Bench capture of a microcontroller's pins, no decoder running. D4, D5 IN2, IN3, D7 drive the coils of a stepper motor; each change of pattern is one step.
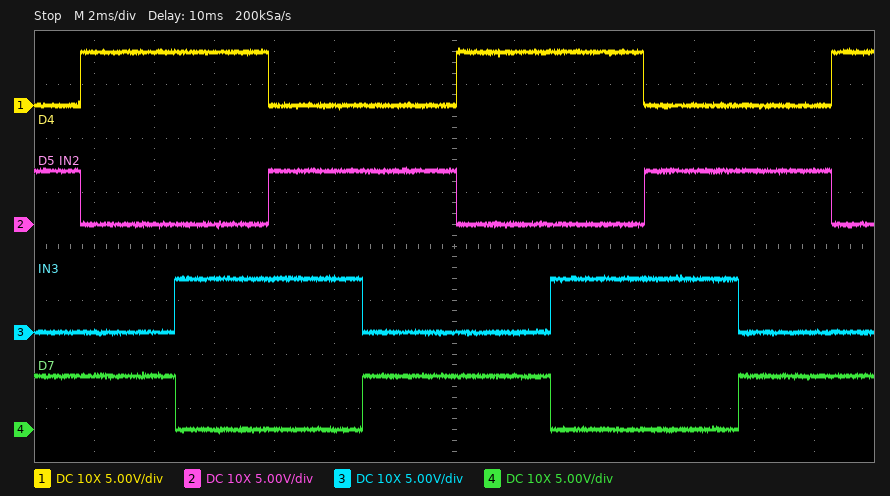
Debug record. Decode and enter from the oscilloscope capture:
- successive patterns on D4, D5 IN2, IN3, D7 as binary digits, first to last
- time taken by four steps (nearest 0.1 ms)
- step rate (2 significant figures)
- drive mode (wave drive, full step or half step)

0101 1001 1010 0110 0101 1001 1010 0110 0101 1001
12.5 ms
320 steps/s
full step
